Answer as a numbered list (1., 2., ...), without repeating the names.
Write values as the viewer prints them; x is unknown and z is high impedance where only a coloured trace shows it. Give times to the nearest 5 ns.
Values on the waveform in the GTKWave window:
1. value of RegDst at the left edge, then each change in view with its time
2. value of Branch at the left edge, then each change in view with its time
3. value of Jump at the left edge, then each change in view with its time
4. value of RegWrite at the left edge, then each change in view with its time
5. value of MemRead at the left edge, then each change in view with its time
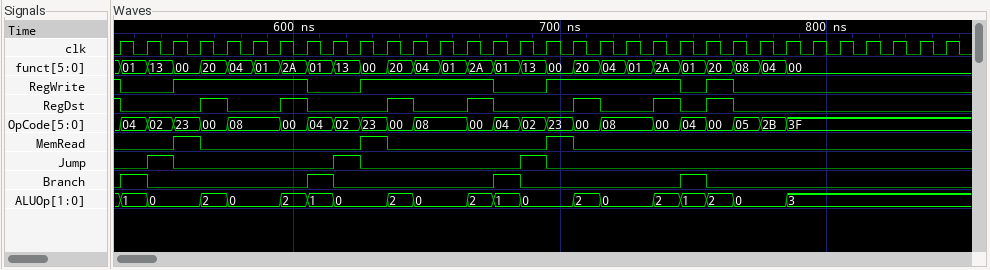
1. 1, 0 at 535 ns, 1 at 565 ns, 0 at 575 ns, 1 at 595 ns, 0 at 605 ns, 1 at 635 ns, 0 at 645 ns, 1 at 665 ns, 0 at 675 ns, 1 at 705 ns, 0 at 715 ns, 1 at 735 ns, 0 at 745 ns, 1 at 755 ns, 0 at 765 ns
2. 0, 1 at 535 ns, 0 at 545 ns, 1 at 605 ns, 0 at 615 ns, 1 at 675 ns, 0 at 685 ns, 1 at 745 ns, 0 at 755 ns
3. 0, 1 at 545 ns, 0 at 555 ns, 1 at 615 ns, 0 at 625 ns, 1 at 685 ns, 0 at 695 ns
4. 1, 0 at 535 ns, 1 at 555 ns, 0 at 605 ns, 1 at 625 ns, 0 at 675 ns, 1 at 695 ns, 0 at 745 ns, 1 at 755 ns, 0 at 765 ns
5. 0, 1 at 555 ns, 0 at 565 ns, 1 at 625 ns, 0 at 635 ns, 1 at 695 ns, 0 at 705 ns
